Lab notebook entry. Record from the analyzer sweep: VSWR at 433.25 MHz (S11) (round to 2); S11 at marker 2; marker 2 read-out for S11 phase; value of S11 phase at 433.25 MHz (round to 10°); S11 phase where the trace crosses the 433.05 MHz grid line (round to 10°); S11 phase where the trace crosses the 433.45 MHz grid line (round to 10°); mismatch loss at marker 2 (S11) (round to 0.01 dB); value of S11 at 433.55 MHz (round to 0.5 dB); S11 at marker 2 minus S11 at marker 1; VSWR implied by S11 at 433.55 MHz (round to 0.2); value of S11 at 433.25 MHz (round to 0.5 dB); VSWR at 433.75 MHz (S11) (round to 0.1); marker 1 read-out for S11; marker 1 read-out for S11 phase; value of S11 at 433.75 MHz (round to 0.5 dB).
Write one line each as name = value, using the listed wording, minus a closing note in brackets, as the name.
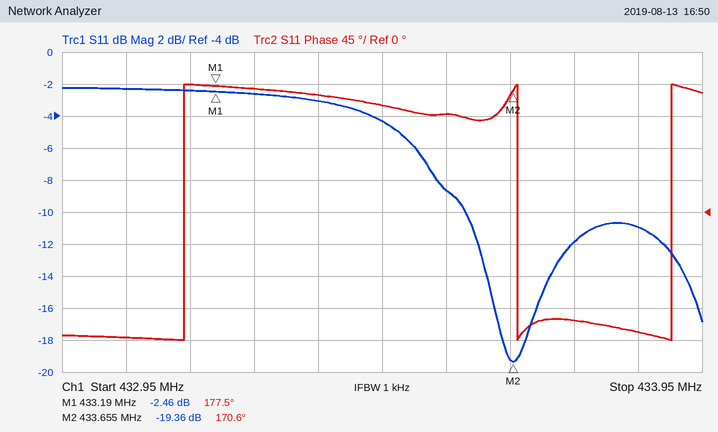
VSWR at 433.25 MHz (S11) = 6
S11 at marker 2 = -19.36 dB
marker 2 read-out for S11 phase = 170.6°
value of S11 phase at 433.25 MHz = 170°
S11 phase where the trace crosses the 433.05 MHz grid line = -180°
S11 phase where the trace crosses the 433.45 MHz grid line = 150°
mismatch loss at marker 2 (S11) = 0.05 dB
value of S11 at 433.55 MHz = -8.5 dB
S11 at marker 2 minus S11 at marker 1 = -16.90 dB
VSWR implied by S11 at 433.55 MHz = 2.2
value of S11 at 433.25 MHz = -2.5 dB
VSWR at 433.75 MHz (S11) = 1.7
marker 1 read-out for S11 = -2.46 dB
marker 1 read-out for S11 phase = 177.5°
value of S11 at 433.75 MHz = -12.0 dB
